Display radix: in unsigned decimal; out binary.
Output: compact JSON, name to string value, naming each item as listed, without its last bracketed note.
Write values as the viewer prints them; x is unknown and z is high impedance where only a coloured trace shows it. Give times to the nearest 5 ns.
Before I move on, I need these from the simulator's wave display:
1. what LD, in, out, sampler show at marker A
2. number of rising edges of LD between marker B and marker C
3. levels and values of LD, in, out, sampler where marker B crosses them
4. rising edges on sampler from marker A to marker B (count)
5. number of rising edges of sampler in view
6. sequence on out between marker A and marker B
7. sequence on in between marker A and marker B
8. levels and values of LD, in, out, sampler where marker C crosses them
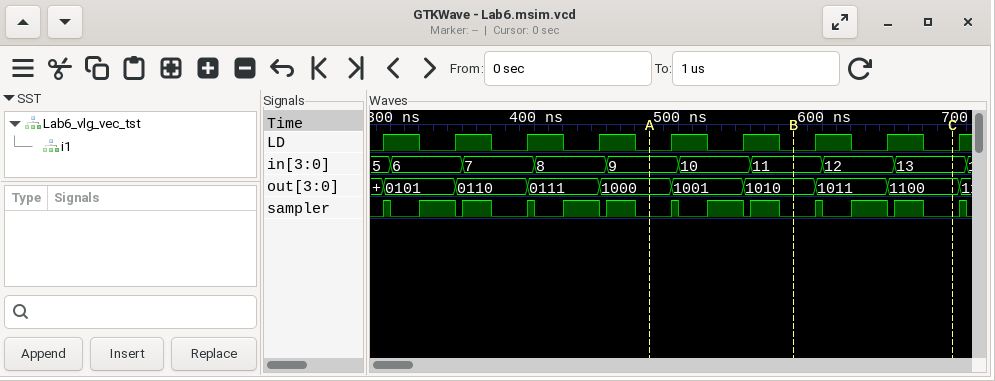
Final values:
{"what LD, in, out, sampler show at marker A": "LD=0, in=9, out=1000, sampler=0", "number of rising edges of LD between marker B and marker C": "2", "levels and values of LD, in, out, sampler where marker B crosses them": "LD=0, in=11, out=1010, sampler=0", "rising edges on sampler from marker A to marker B": "3", "number of rising edges of sampler in view": "13", "sequence on out between marker A and marker B": "1000, 1001, 1010", "sequence on in between marker A and marker B": "9, 10, 11", "levels and values of LD, in, out, sampler where marker C crosses them": "LD=0, in=13, out=1100, sampler=0"}
